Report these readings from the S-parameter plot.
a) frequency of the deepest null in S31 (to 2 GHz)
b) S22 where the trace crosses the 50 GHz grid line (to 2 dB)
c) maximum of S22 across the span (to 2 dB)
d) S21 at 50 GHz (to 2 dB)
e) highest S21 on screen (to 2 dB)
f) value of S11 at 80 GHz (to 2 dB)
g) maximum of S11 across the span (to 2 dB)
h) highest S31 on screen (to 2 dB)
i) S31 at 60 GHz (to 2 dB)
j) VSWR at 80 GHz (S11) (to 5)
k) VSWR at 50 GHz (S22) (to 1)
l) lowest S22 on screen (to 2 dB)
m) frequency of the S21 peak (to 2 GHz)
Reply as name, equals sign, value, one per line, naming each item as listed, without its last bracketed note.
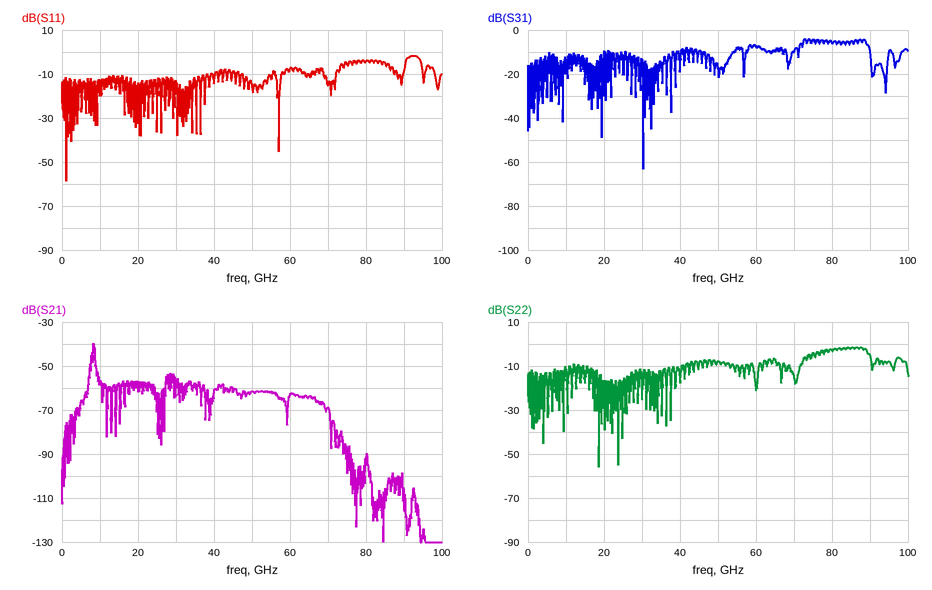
frequency of the deepest null in S31 = 30 GHz
S22 where the trace crosses the 50 GHz grid line = -8 dB
maximum of S22 across the span = -2 dB
S21 at 50 GHz = -62 dB
highest S21 on screen = -40 dB
value of S11 at 80 GHz = -4 dB
maximum of S11 across the span = -2 dB
highest S31 on screen = -4 dB
S31 at 60 GHz = -8 dB
VSWR at 80 GHz (S11) = 5
VSWR at 50 GHz (S22) = 2
lowest S22 on screen = -56 dB
frequency of the S21 peak = 8 GHz
